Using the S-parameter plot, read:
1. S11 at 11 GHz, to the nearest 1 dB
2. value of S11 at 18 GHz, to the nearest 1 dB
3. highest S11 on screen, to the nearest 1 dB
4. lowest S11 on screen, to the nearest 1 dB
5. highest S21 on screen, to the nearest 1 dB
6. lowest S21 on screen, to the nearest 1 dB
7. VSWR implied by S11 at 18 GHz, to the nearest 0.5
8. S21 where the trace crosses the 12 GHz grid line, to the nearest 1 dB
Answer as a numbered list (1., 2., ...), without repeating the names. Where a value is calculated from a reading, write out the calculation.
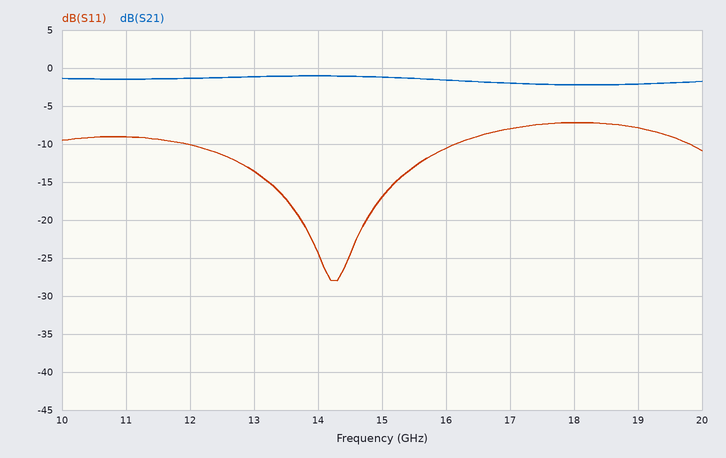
1. -9 dB
2. -7 dB
3. -7 dB
4. -28 dB
5. -1 dB
6. -2 dB
7. |Γ| = 10^(-7/20) = 0.4467; VSWR = (1 + 0.4467)/(1 − 0.4467) ≈ 2.61, so 2.5 to the nearest 0.5
8. -1 dB
